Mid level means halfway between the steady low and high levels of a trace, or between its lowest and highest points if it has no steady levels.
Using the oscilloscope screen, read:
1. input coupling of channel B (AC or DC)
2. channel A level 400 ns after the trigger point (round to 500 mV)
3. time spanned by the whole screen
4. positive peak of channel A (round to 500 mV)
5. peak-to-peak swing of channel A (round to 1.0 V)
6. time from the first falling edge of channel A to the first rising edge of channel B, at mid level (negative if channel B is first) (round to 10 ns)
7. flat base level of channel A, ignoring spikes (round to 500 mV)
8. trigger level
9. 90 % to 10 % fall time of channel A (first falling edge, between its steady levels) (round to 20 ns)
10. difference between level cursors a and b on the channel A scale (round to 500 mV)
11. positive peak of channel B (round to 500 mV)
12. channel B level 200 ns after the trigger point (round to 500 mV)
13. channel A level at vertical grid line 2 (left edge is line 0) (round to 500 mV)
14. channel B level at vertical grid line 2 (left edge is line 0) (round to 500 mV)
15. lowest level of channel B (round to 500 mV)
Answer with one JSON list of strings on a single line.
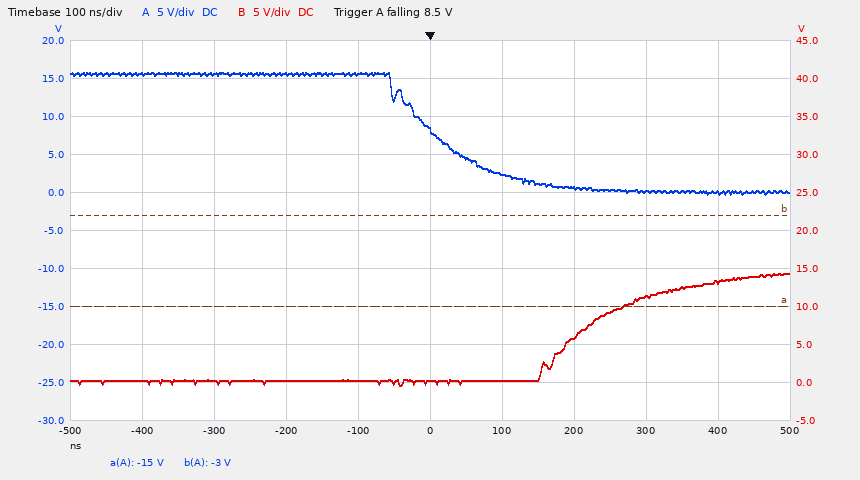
["DC", "0.0 V", "1 µs", "16.0 V", "16.0 V", "+210 ns", "0.0 V", "8.5 V", "180 ns", "12.0 V", "14.5 V", "6.0 V", "15.5 V", "0.0 V", "-500 mV"]
